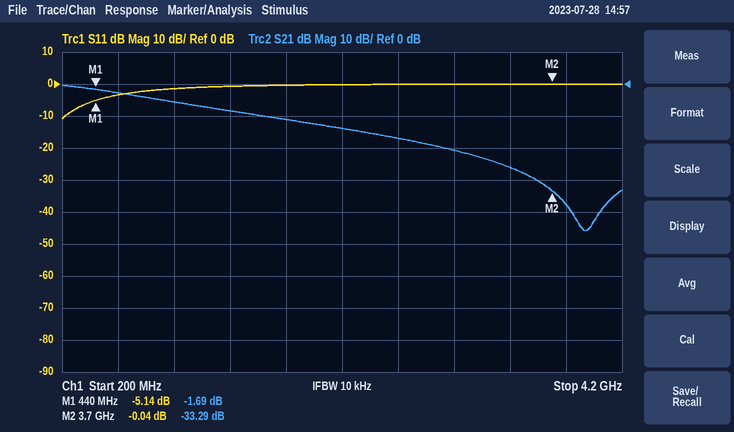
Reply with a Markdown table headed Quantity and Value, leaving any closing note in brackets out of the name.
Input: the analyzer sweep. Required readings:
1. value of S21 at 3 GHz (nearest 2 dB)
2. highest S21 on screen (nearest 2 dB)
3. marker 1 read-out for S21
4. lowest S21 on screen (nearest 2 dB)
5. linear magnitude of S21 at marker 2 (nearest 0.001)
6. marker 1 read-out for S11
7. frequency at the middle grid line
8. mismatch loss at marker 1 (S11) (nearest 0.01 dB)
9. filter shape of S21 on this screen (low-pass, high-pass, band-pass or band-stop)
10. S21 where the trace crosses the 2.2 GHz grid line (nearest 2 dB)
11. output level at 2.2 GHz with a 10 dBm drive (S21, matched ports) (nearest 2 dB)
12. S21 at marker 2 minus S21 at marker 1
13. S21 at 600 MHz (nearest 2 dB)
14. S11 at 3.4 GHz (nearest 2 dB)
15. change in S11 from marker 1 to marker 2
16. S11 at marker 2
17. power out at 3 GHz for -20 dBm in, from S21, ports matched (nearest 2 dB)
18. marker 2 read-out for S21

| Quantity | Value |
|---|---|
| value of S21 at 3 GHz | -20 dB |
| highest S21 on screen | 0 dB |
| marker 1 read-out for S21 | -1.69 dB |
| lowest S21 on screen | -46 dB |
| linear magnitude of S21 at marker 2 | 0.022 |
| marker 1 read-out for S11 | -5.14 dB |
| frequency at the middle grid line | 2.2 GHz |
| mismatch loss at marker 1 (S11) | 1.59 dB |
| filter shape of S21 on this screen | low-pass |
| S21 where the trace crosses the 2.2 GHz grid line | -14 dB |
| output level at 2.2 GHz with a 10 dBm drive (S21, matched ports) | -4 dBm |
| S21 at marker 2 minus S21 at marker 1 | -31.60 dB |
| S21 at 600 MHz | -2 dB |
| S11 at 3.4 GHz | 0 dB |
| change in S11 from marker 1 to marker 2 | 5.10 dB |
| S11 at marker 2 | -0.04 dB |
| power out at 3 GHz for -20 dBm in, from S21, ports matched | -40 dBm |
| marker 2 read-out for S21 | -33.29 dB |
